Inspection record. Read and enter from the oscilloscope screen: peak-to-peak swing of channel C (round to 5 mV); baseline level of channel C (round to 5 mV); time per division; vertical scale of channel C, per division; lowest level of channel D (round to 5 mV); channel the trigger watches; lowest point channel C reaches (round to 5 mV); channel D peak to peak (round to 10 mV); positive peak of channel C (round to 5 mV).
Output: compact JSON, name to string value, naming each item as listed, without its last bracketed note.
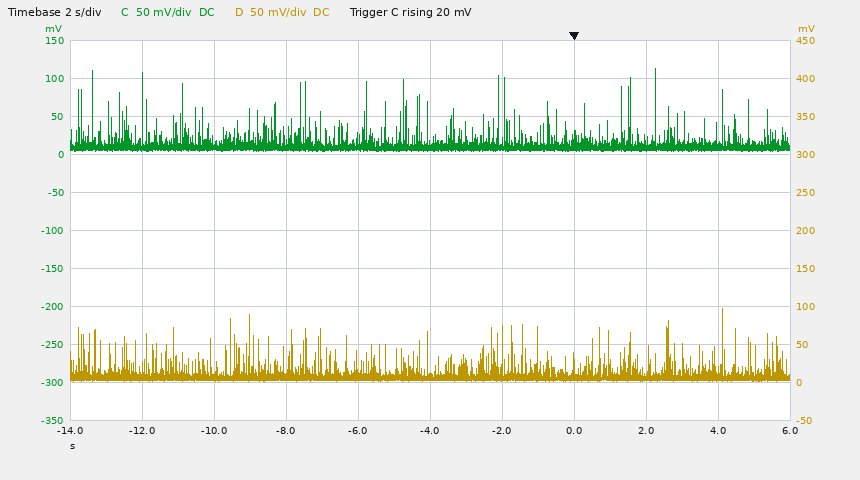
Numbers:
{"peak-to-peak swing of channel C": "110 mV", "baseline level of channel C": "10 mV", "time per division": "2 s", "vertical scale of channel C, per division": "50 mV", "lowest level of channel D": "0 mV", "channel the trigger watches": "channel C", "lowest point channel C reaches": "5 mV", "channel D peak to peak": "100 mV", "positive peak of channel C": "115 mV"}
